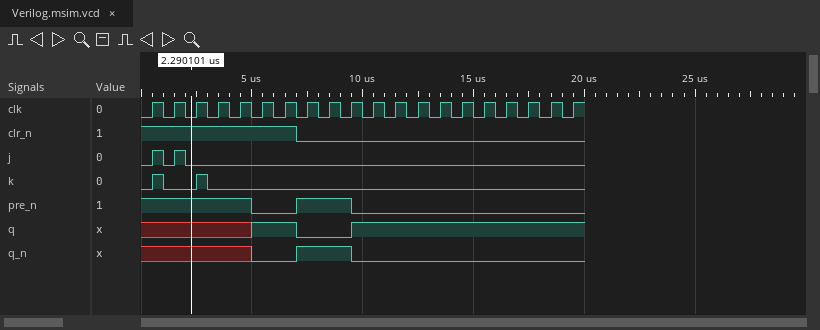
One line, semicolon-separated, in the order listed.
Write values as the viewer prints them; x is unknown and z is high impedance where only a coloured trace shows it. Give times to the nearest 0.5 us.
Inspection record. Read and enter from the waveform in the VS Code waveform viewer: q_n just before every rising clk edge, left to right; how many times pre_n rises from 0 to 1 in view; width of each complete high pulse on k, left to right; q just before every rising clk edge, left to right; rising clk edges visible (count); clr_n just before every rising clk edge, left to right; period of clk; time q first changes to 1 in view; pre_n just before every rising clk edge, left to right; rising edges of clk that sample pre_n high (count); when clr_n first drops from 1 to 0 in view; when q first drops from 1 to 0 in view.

x x x x x 0 0 1 1 1 0 0 0 0 0 0 0 0 0 0; 1; 0.5 us, 0.5 us; x x x x x 1 1 0 0 0 1 1 1 1 1 1 1 1 1 1; 20; 1 1 1 1 1 1 1 0 0 0 0 0 0 0 0 0 0 0 0 0; 1 us; 5 us; 1 1 1 1 1 0 0 1 1 1 0 0 0 0 0 0 0 0 0 0; 8; 7 us; 7 us
